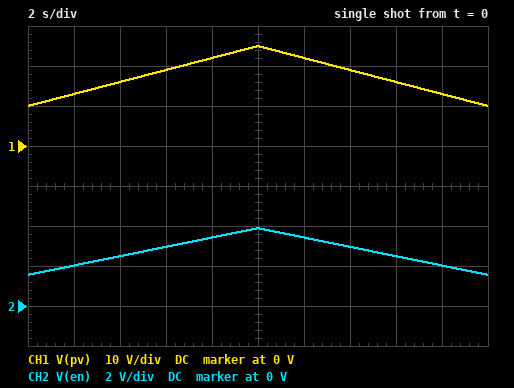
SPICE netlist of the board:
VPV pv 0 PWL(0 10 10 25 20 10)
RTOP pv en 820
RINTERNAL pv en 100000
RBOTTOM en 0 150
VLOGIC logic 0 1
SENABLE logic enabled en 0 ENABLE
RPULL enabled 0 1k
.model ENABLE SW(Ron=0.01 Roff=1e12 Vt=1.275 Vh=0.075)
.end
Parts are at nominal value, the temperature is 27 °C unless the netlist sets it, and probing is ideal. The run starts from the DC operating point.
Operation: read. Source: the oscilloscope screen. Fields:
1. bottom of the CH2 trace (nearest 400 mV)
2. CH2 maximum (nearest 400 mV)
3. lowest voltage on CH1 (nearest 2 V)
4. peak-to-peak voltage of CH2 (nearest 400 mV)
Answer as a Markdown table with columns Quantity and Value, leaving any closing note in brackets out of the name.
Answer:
| Quantity | Value |
|---|---|
| bottom of the CH2 trace | 1.6 V |
| CH2 maximum | 4.0 V |
| lowest voltage on CH1 | 10 V |
| peak-to-peak voltage of CH2 | 2.4 V |
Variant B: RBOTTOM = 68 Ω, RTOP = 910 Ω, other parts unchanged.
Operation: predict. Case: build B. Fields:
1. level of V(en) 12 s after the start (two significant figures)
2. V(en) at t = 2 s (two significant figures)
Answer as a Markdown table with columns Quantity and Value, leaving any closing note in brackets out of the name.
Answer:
| Quantity | Value |
|---|---|
| level of V(en) 12 s after the start | 1.5 V |
| V(en) at t = 2 s | 910 mV |
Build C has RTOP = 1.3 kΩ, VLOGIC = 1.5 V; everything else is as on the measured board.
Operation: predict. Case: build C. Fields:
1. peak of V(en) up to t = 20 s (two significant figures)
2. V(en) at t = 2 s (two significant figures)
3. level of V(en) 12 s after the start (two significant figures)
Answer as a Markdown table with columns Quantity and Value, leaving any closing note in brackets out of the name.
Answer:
| Quantity | Value |
|---|---|
| peak of V(en) up to t = 20 s | 2.6 V |
| V(en) at t = 2 s | 1.4 V |
| level of V(en) 12 s after the start | 2.3 V |
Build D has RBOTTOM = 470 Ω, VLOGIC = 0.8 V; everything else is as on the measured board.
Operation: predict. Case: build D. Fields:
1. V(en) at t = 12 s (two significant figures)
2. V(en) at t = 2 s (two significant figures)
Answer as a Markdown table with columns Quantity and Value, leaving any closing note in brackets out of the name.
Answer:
| Quantity | Value |
|---|---|
| V(en) at t = 12 s | 8.1 V |
| V(en) at t = 2 s | 4.8 V |
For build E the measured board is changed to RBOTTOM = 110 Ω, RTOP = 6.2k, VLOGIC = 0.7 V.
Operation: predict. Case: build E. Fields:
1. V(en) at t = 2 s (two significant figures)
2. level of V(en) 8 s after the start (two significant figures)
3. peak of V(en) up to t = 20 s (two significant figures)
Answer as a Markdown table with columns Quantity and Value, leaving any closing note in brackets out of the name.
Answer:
| Quantity | Value |
|---|---|
| V(en) at t = 2 s | 240 mV |
| level of V(en) 8 s after the start | 410 mV |
| peak of V(en) up to t = 20 s | 460 mV |
